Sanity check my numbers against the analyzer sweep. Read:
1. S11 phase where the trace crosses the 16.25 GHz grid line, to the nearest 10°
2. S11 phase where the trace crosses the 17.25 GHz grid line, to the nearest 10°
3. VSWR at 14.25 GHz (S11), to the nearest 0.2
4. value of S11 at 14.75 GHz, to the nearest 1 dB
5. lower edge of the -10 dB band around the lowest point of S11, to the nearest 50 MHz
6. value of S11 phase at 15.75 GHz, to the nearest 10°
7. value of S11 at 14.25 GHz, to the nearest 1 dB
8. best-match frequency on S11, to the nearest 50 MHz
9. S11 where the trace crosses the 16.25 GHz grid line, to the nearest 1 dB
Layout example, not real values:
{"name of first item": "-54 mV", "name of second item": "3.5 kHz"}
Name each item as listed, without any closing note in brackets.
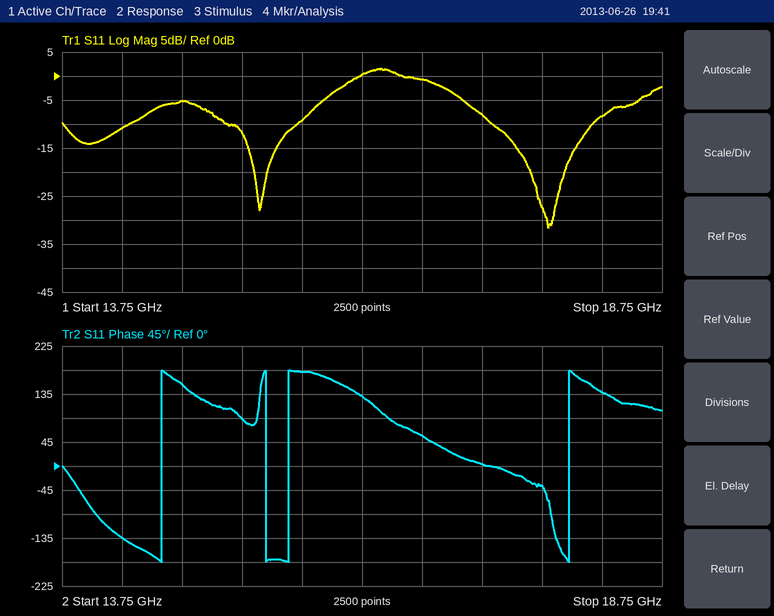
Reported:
{"S11 phase where the trace crosses the 16.25 GHz grid line, to the nearest 10°": "130°", "S11 phase where the trace crosses the 17.25 GHz grid line, to the nearest 10°": "0°", "VSWR at 14.25 GHz (S11), to the nearest 0.2": "1.8", "value of S11 at 14.75 GHz, to the nearest 1 dB": "-5 dB", "lower edge of the -10 dB band around the lowest point of S11, to the nearest 50 MHz": "17.35 GHz", "value of S11 phase at 15.75 GHz, to the nearest 10°": "180°", "value of S11 at 14.25 GHz, to the nearest 1 dB": "-11 dB", "best-match frequency on S11, to the nearest 50 MHz": "17.80 GHz", "S11 where the trace crosses the 16.25 GHz grid line, to the nearest 1 dB": "0 dB"}
